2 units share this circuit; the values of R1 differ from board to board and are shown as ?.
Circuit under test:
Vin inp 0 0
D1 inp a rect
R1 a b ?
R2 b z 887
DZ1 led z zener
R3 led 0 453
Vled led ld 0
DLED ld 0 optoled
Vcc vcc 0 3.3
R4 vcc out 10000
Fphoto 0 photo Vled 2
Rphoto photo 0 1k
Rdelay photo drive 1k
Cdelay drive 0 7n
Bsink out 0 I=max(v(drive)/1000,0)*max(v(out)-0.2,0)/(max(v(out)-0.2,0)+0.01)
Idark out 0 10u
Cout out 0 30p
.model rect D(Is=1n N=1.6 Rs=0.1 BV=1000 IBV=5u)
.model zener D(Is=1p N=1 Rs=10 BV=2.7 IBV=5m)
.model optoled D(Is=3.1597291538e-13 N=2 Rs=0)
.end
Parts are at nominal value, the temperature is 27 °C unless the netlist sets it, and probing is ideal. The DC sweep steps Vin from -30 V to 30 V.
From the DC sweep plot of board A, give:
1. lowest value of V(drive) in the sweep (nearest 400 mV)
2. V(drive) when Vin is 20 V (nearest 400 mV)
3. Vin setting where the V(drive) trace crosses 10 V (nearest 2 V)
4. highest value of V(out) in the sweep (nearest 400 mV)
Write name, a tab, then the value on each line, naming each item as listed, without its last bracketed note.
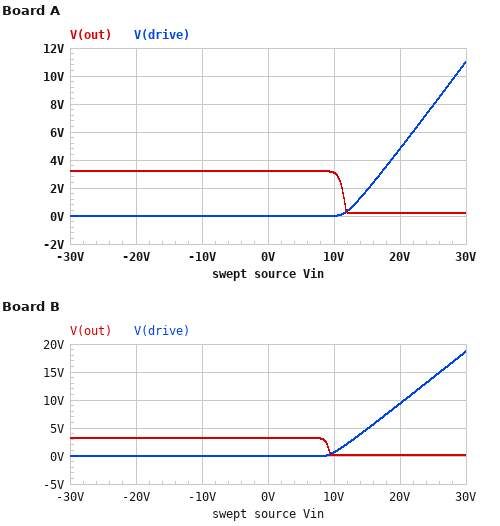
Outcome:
lowest value of V(drive) in the sweep	0 V
V(drive) when Vin is 20 V	4.8 V
Vin setting where the V(drive) trace crosses 10 V	28 V
highest value of V(out) in the sweep	3.2 V
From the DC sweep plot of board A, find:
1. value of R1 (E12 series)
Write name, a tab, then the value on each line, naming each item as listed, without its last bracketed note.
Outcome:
value of R1	2.2 kΩ
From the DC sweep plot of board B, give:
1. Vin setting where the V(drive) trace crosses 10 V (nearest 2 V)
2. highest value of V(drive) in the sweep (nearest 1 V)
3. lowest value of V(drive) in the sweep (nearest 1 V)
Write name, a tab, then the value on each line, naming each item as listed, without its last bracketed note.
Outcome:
Vin setting where the V(drive) trace crosses 10 V	20 V
highest value of V(drive) in the sweep	19 V
lowest value of V(drive) in the sweep	0 V
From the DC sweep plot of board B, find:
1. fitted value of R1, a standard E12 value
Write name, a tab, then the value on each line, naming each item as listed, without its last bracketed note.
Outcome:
fitted value of R1, a standard E12 value	1.2 kΩ
